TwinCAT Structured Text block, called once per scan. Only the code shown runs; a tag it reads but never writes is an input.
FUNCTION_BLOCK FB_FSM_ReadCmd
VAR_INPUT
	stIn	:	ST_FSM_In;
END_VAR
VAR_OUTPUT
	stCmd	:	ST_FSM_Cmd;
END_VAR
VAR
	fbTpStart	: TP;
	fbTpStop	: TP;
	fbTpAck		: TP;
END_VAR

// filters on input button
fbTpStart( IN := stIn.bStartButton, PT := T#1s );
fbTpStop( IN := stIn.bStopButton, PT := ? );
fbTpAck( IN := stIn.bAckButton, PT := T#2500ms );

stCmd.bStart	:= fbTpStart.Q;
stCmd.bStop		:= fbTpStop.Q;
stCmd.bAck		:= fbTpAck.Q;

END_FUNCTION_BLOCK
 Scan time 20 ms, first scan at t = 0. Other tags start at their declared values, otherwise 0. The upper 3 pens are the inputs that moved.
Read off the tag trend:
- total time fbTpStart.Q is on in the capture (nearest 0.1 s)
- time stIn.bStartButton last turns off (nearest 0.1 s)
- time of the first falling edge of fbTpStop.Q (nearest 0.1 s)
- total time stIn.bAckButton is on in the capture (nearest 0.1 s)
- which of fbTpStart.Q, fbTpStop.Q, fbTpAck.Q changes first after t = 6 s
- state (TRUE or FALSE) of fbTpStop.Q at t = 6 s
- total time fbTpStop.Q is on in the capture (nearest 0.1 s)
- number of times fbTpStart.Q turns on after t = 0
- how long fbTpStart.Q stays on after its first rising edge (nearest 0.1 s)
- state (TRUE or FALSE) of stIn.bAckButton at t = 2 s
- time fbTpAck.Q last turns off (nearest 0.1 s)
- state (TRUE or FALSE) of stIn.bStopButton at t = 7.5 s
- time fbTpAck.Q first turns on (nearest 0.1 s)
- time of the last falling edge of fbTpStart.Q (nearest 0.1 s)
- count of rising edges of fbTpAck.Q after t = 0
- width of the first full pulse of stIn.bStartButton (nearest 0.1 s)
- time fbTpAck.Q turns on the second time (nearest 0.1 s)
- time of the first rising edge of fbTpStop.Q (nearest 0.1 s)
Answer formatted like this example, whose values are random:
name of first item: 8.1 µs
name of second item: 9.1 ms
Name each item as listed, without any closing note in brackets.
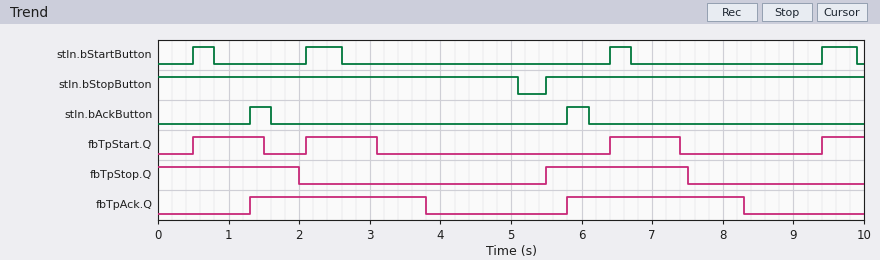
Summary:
total time fbTpStart.Q is on in the capture: 3.6 s
time stIn.bStartButton last turns off: 9.9 s
time of the first falling edge of fbTpStop.Q: 2.0 s
total time stIn.bAckButton is on in the capture: 0.6 s
which of fbTpStart.Q, fbTpStop.Q, fbTpAck.Q changes first after t = 6 s: fbTpStart.Q
state (TRUE or FALSE) of fbTpStop.Q at t = 6 s: TRUE
total time fbTpStop.Q is on in the capture: 4.0 s
number of times fbTpStart.Q turns on after t = 0: 4
how long fbTpStart.Q stays on after its first rising edge: 1.0 s
state (TRUE or FALSE) of stIn.bAckButton at t = 2 s: FALSE
time fbTpAck.Q last turns off: 8.3 s
state (TRUE or FALSE) of stIn.bStopButton at t = 7.5 s: TRUE
time fbTpAck.Q first turns on: 1.3 s
time of the last falling edge of fbTpStart.Q: 7.4 s
count of rising edges of fbTpAck.Q after t = 0: 2
width of the first full pulse of stIn.bStartButton: 0.3 s
time fbTpAck.Q turns on the second time: 5.8 s
time of the first rising edge of fbTpStop.Q: 5.5 s
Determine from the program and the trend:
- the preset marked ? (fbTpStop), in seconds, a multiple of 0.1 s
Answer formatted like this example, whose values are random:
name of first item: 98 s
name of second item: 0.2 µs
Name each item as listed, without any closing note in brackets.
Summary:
the preset marked ? (fbTpStop), in seconds, a multiple of 0.1 s: 2.0 s
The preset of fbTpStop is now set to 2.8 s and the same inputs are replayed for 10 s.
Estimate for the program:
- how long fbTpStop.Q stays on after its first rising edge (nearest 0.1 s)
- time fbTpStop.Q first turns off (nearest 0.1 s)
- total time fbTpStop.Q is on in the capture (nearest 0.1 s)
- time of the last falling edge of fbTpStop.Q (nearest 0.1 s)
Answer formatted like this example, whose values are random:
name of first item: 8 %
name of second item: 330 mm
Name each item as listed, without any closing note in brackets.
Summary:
how long fbTpStop.Q stays on after its first rising edge: 2.8 s
time fbTpStop.Q first turns off: 2.8 s
total time fbTpStop.Q is on in the capture: 5.6 s
time of the last falling edge of fbTpStop.Q: 8.3 s
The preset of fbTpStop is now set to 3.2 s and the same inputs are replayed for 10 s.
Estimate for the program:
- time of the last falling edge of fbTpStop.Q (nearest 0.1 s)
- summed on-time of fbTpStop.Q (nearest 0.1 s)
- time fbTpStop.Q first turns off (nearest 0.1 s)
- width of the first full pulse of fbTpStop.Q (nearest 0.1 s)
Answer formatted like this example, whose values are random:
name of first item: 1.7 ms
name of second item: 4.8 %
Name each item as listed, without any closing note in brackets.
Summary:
time of the last falling edge of fbTpStop.Q: 8.7 s
summed on-time of fbTpStop.Q: 6.4 s
time fbTpStop.Q first turns off: 3.2 s
width of the first full pulse of fbTpStop.Q: 3.2 s
